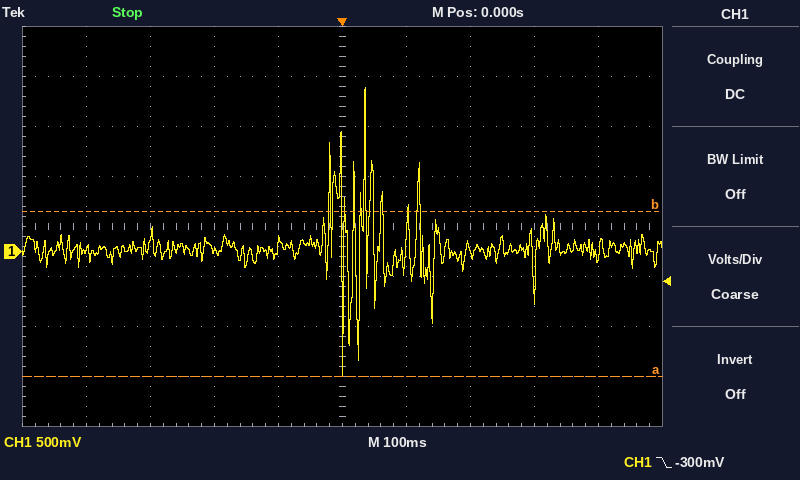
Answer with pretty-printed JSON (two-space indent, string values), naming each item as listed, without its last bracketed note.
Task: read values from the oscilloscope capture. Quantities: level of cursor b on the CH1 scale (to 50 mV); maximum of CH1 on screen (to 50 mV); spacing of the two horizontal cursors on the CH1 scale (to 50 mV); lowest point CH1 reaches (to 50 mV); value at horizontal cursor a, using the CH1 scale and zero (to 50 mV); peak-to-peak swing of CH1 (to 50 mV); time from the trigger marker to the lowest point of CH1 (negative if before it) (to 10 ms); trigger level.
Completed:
{
  "level of cursor b on the CH1 scale": "400 mV",
  "maximum of CH1 on screen": "1.65 V",
  "spacing of the two horizontal cursors on the CH1 scale": "1.65 V",
  "lowest point CH1 reaches": "-1.25 V",
  "value at horizontal cursor a, using the CH1 scale and zero": "-1.25 V",
  "peak-to-peak swing of CH1": "2.90 V",
  "time from the trigger marker to the lowest point of CH1 (negative if before it)": "0 ms",
  "trigger level": "-300 mV"
}
